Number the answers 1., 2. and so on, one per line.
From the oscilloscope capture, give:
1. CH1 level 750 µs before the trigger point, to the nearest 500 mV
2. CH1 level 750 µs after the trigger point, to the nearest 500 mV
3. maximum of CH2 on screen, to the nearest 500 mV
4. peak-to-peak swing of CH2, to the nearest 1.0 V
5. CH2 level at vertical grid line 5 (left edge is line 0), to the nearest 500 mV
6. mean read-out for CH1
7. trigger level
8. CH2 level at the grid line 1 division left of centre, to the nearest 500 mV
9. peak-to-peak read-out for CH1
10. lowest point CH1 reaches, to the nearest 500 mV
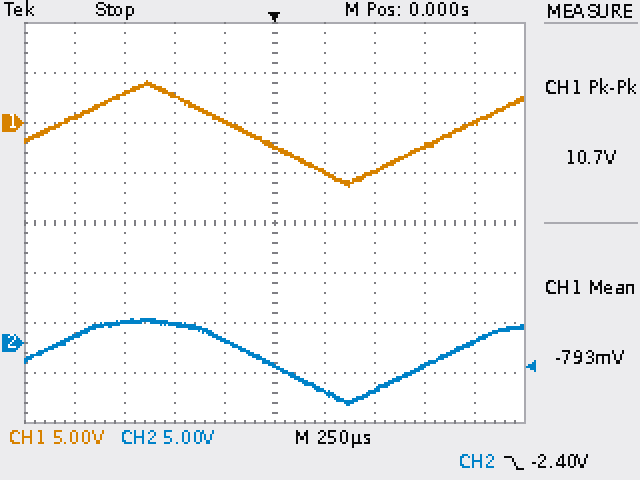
1. 3.0 V
2. -2.5 V
3. 2.5 V
4. 9.0 V
5. -2.5 V
6. -793 mV
7. -2.40 V
8. 500 mV
9. 10.7 V
10. -6.5 V
